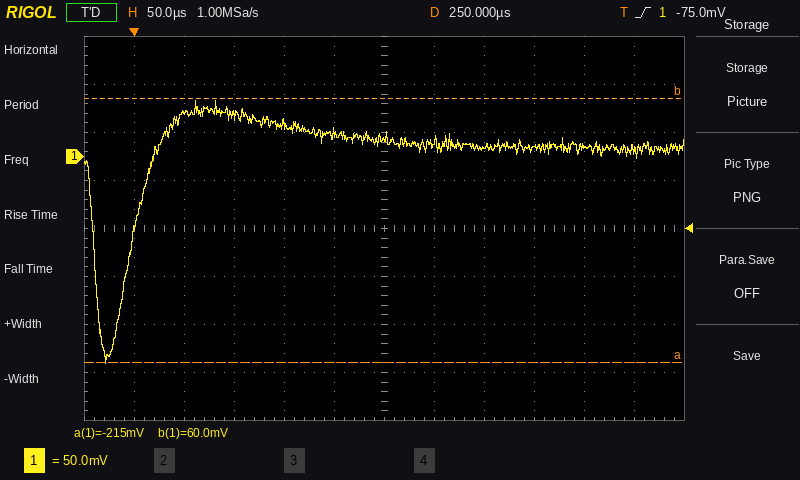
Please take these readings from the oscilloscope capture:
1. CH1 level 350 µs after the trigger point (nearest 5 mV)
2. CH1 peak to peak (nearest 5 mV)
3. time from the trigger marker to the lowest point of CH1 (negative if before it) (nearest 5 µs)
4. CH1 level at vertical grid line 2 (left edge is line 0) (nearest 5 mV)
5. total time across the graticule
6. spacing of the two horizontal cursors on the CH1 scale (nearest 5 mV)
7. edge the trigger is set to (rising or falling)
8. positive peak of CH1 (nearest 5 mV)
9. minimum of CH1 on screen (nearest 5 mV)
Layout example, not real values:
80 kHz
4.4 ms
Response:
10 mV
275 mV
-30 µs
45 mV
600 µs
275 mV
rising
60 mV
-215 mV
